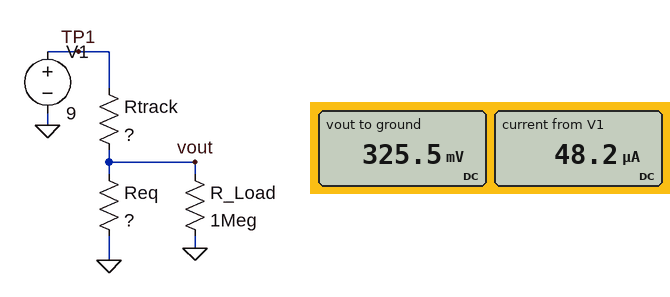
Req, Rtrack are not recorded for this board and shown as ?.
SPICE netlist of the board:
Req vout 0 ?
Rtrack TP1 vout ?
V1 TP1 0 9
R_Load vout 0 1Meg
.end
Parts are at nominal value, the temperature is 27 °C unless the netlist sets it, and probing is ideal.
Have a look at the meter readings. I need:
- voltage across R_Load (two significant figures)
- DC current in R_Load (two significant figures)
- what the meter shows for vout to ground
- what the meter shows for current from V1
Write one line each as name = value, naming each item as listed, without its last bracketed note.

voltage across R_Load = 330 mV
DC current in R_Load = 330 nA
what the meter shows for vout to ground = 325.5 mV
what the meter shows for current from V1 = 48.2 µA
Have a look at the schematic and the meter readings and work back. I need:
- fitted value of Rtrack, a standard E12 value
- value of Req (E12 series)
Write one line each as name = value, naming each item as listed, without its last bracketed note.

fitted value of Rtrack, a standard E12 value = 180 kΩ
value of Req = 6.8 kΩ
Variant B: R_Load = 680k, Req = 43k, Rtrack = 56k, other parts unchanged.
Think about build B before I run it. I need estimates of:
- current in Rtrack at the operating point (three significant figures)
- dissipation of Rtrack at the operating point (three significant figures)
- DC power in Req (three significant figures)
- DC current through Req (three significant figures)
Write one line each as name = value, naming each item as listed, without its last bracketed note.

current in Rtrack at the operating point = 93.3 µA
dissipation of Rtrack at the operating point = 488 µW
DC power in Req = 331 µW
DC current through Req = 87.8 µA
